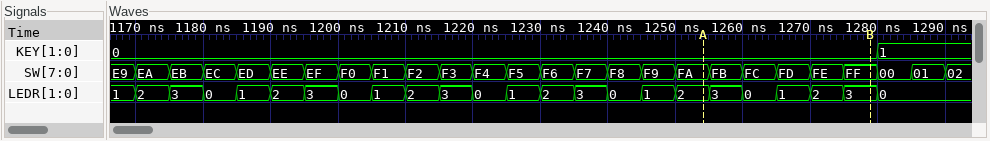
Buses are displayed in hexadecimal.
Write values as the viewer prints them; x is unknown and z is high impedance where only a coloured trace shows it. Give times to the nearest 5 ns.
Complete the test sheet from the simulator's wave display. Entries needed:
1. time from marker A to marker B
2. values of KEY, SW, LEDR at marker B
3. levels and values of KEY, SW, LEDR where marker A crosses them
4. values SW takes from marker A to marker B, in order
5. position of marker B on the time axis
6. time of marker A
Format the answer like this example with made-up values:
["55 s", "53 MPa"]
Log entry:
["25 ns", "KEY=0, SW=FF, LEDR=3", "KEY=0, SW=FA, LEDR=2", "FA, FB, FC, FD, FE, FF", "1280 ns", "1255 ns"]
